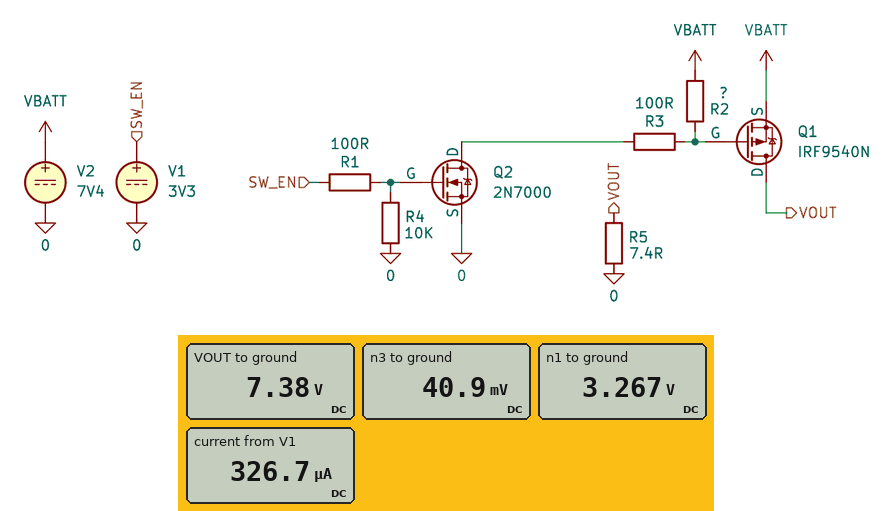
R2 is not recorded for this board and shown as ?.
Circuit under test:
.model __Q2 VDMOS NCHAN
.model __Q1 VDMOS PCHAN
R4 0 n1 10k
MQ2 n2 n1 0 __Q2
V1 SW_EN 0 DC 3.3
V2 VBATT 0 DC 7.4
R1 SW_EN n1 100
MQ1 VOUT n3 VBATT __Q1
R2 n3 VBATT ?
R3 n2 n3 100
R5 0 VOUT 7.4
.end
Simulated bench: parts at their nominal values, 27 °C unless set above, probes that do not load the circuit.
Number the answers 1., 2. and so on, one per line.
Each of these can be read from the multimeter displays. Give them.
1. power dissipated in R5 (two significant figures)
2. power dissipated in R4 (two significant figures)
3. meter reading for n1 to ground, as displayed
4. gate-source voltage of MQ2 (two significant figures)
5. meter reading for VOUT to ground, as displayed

1. 7.4 W
2. 1.1 mW
3. 3.267 V
4. 3.3 V
5. 7.38 V
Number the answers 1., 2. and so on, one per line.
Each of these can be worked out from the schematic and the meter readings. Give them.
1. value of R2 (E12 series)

1. 18 kΩ
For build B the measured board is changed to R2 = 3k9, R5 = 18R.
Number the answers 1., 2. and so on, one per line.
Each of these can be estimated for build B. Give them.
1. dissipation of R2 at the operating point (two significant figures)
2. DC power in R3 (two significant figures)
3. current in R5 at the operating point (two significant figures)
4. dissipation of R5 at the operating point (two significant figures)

1. 13 mW
2. 340 µW
3. 410 mA
4. 3.0 W
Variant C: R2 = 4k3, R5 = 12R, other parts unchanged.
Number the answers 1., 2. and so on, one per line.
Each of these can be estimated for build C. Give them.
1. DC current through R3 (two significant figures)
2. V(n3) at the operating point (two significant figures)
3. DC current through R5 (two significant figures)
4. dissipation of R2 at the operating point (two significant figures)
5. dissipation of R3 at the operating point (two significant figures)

1. 1.7 mA
2. 170 mV
3. 620 mA
4. 12 mW
5. 280 µW
